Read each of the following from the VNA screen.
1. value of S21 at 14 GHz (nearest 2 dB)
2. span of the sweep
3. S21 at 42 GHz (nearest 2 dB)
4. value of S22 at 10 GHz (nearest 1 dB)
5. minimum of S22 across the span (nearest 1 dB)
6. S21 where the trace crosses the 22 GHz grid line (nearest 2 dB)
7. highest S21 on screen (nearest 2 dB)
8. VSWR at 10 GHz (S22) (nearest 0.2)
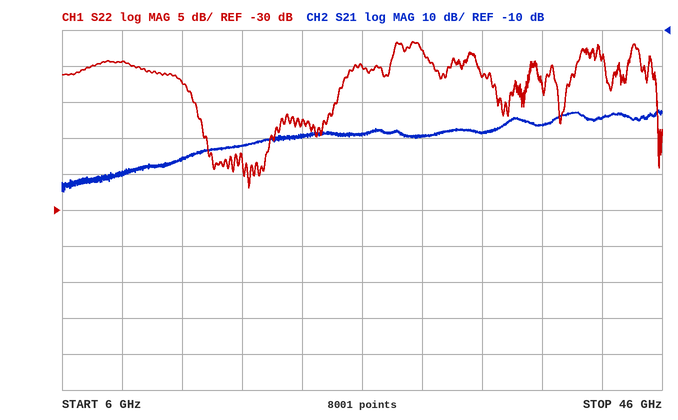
-46 dB
40 GHz
-34 dB
-9 dB
-27 dB
-40 dB
-32 dB
2.0
